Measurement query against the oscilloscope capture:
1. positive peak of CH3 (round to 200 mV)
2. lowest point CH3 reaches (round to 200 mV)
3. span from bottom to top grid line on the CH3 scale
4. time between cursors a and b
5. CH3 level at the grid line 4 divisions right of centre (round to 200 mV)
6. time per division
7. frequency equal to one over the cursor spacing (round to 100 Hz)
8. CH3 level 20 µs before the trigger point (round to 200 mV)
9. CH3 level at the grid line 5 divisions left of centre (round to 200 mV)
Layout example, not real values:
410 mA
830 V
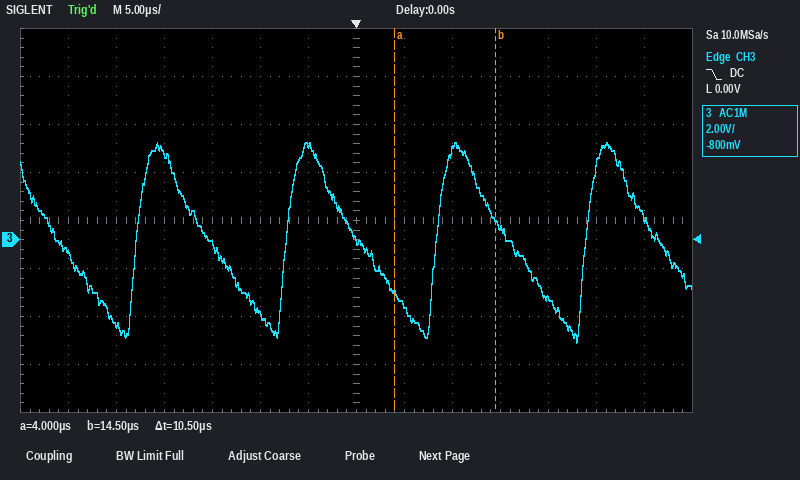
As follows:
4.0 V
-4.2 V
16 V
10.5 µs
-2.4 V
5 µs
95.2 kHz
3.6 V
-3.6 V
